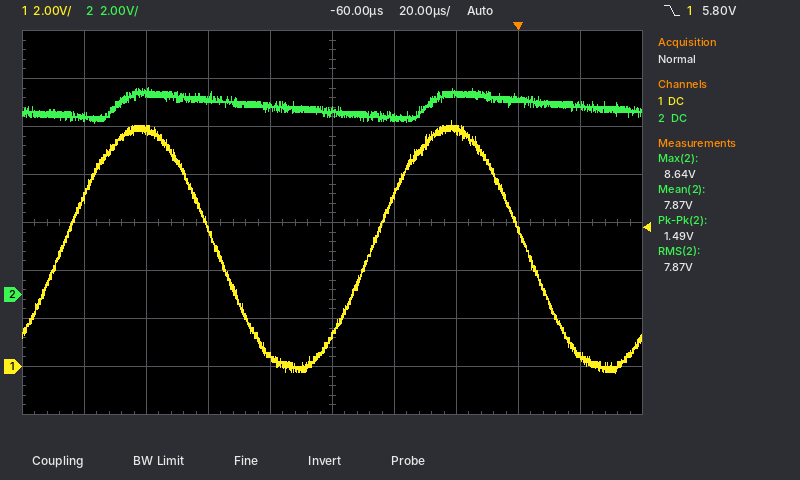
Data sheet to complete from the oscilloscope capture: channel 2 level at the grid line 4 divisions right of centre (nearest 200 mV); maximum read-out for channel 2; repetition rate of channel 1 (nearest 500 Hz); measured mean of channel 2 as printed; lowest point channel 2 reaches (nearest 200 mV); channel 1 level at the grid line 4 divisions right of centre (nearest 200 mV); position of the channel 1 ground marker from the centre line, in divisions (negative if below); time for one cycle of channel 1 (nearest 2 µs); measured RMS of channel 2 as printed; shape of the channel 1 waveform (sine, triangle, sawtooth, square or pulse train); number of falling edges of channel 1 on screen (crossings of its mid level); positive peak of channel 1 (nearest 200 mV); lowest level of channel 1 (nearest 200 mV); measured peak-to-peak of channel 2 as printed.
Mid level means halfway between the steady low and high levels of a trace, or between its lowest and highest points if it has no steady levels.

7.8 V
8.64 V
10.0 kHz
7.87 V
7.2 V
400 mV
-3.0 div
100 µs
7.87 V
sine
2
10.2 V
-200 mV
1.49 V
